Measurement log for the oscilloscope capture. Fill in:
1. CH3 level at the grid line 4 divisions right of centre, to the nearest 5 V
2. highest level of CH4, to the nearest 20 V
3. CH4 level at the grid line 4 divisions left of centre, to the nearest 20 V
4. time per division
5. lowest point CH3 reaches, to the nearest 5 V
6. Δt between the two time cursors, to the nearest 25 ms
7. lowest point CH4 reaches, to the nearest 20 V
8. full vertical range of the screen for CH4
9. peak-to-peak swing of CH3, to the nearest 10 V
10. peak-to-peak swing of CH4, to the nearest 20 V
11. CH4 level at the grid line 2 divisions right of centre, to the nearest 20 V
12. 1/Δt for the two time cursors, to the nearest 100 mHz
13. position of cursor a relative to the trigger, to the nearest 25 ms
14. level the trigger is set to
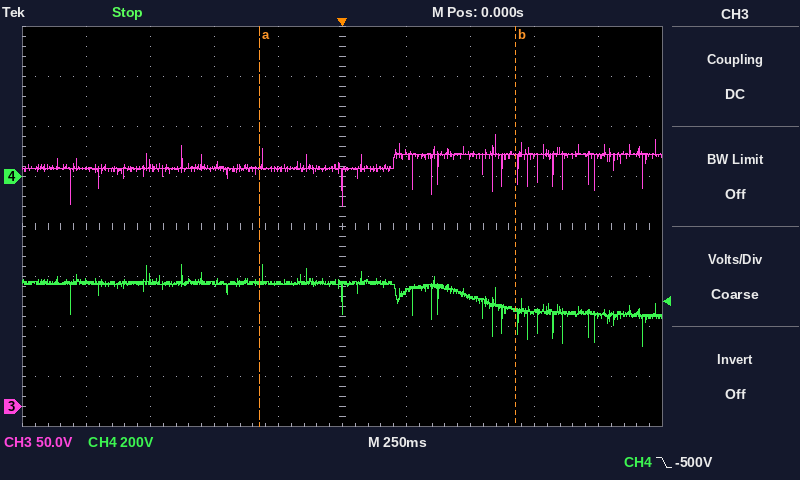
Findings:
250 V
-360 V
-420 V
250 ms
200 V
1.000 s
-680 V
1.6 kV
70 V
320 V
-480 V
1.0 Hz
-325 ms
-500 V
